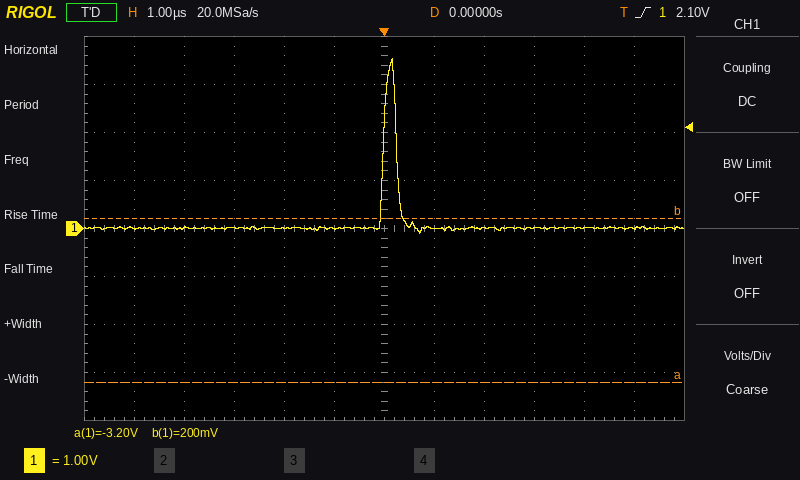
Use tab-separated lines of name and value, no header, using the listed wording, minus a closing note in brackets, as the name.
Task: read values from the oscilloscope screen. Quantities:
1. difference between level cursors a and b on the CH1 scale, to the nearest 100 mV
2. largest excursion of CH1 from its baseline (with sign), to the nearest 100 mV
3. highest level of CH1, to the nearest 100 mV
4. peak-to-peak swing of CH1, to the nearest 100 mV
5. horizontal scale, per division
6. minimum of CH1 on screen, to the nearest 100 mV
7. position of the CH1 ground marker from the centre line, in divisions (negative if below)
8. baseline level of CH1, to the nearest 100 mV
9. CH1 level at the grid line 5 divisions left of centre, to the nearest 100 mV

difference between level cursors a and b on the CH1 scale, to the nearest 100 mV	3.4 V
largest excursion of CH1 from its baseline (with sign), to the nearest 100 mV	+3.5 V
highest level of CH1, to the nearest 100 mV	3.5 V
peak-to-peak swing of CH1, to the nearest 100 mV	3.6 V
horizontal scale, per division	1 µs
minimum of CH1 on screen, to the nearest 100 mV	-100 mV
position of the CH1 ground marker from the centre line, in divisions	0.0 div
baseline level of CH1, to the nearest 100 mV	0.0 V
CH1 level at the grid line 5 divisions left of centre, to the nearest 100 mV	0.0 V
